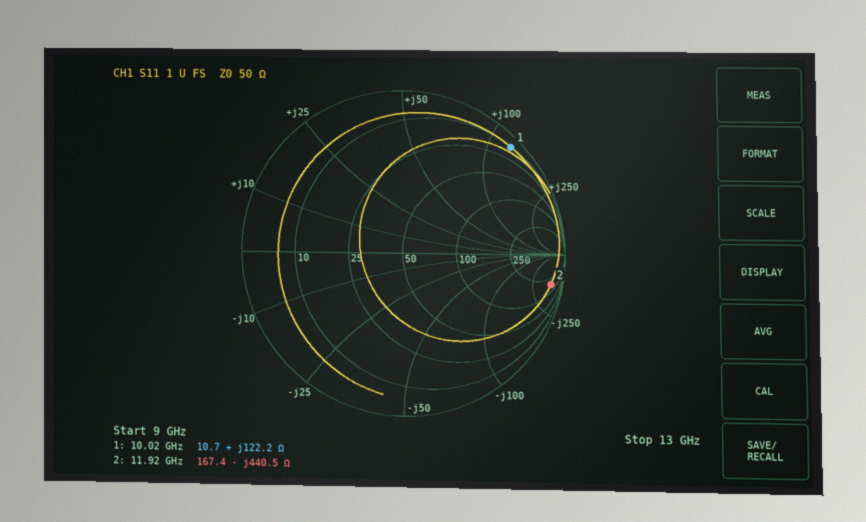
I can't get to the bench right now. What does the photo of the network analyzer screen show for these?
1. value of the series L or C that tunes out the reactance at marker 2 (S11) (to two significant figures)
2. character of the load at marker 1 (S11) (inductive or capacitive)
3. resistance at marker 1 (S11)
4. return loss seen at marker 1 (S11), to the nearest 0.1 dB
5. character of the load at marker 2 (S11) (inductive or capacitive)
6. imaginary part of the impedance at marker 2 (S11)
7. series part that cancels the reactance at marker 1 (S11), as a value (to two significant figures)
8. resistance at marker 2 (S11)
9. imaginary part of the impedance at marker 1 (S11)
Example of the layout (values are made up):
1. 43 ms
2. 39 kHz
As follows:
1. 5.9 nH
2. inductive
3. 10.7 Ω
4. 0.5 dB
5. capacitive
6. -440.5 Ω
7. 130 fF
8. 167.4 Ω
9. +122.2 Ω
